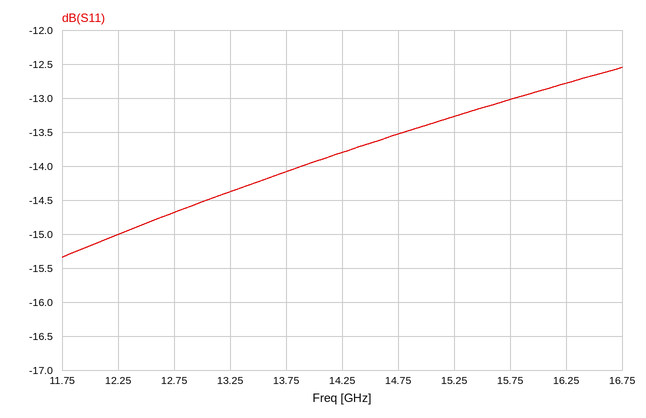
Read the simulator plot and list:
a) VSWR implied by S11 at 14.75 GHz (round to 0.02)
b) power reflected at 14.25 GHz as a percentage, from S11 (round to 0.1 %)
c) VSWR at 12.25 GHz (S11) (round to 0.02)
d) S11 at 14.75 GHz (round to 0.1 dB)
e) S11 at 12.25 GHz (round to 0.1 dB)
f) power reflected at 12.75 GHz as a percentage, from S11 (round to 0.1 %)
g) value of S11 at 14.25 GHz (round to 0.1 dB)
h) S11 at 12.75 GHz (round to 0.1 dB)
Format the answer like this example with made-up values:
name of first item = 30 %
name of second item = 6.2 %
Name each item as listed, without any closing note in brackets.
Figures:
VSWR implied by S11 at 14.75 GHz = 1.54
power reflected at 14.25 GHz as a percentage, from S11 = 4.2 %
VSWR at 12.25 GHz (S11) = 1.44
S11 at 14.75 GHz = -13.5 dB
S11 at 12.25 GHz = -15.0 dB
power reflected at 12.75 GHz as a percentage, from S11 = 3.4 %
value of S11 at 14.25 GHz = -13.8 dB
S11 at 12.75 GHz = -14.7 dB
